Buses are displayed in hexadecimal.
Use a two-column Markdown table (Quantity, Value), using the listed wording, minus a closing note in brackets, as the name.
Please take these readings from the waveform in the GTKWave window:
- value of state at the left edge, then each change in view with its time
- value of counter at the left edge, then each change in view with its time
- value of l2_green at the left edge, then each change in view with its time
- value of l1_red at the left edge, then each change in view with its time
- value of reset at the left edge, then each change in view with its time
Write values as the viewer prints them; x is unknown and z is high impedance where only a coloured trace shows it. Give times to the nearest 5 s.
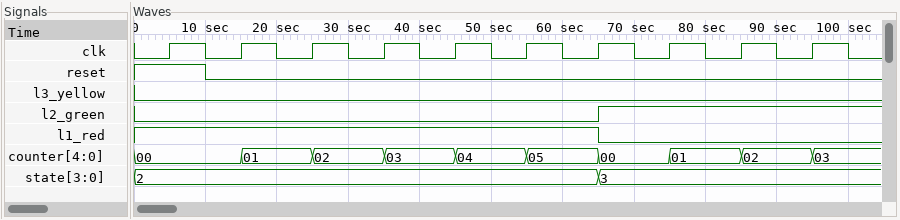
| Quantity | Value |
|---|---|
| value of state at the left edge, then each change in view with its time | 2, 3 at 65 s |
| value of counter at the left edge, then each change in view with its time | 00, 01 at 15 s, 02 at 25 s, 03 at 35 s, 04 at 45 s, 05 at 55 s, 00 at 65 s, 01 at 75 s, 02 at 85 s, 03 at 95 s |
| value of l2_green at the left edge, then each change in view with its time | 0, 1 at 65 s |
| value of l1_red at the left edge, then each change in view with its time | 1, 0 at 65 s |
| value of reset at the left edge, then each change in view with its time | 1, 0 at 10 s |
